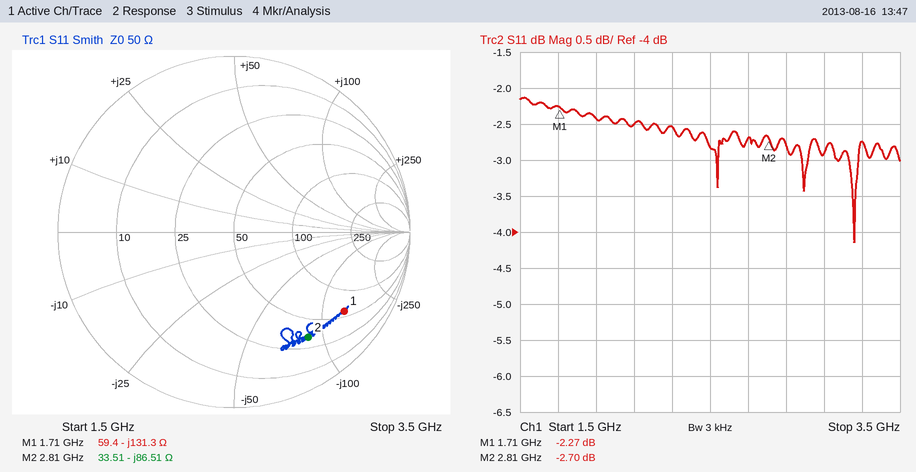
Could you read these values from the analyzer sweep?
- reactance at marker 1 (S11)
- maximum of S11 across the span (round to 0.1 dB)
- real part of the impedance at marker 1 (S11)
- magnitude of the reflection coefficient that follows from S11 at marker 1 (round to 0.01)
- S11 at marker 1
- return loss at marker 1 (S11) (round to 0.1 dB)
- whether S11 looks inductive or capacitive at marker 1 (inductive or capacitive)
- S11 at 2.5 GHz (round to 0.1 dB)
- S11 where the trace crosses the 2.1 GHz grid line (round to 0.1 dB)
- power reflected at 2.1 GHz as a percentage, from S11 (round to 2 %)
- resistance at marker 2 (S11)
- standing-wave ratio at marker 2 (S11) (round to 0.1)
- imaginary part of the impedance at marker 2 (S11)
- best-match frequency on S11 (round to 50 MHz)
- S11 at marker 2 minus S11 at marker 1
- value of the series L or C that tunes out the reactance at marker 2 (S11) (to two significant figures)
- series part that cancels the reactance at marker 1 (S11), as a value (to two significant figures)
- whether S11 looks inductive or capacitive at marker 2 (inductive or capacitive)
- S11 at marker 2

-131.3 Ω
-2.1 dB
59.4 Ω
0.77
-2.27 dB
2.3 dB
capacitive
-2.8 dB
-2.5 dB
56 %
33.51 Ω
6.5
-86.51 Ω
3.25 GHz
-0.43 dB
4.9 nH
12 nH
capacitive
-2.70 dB
